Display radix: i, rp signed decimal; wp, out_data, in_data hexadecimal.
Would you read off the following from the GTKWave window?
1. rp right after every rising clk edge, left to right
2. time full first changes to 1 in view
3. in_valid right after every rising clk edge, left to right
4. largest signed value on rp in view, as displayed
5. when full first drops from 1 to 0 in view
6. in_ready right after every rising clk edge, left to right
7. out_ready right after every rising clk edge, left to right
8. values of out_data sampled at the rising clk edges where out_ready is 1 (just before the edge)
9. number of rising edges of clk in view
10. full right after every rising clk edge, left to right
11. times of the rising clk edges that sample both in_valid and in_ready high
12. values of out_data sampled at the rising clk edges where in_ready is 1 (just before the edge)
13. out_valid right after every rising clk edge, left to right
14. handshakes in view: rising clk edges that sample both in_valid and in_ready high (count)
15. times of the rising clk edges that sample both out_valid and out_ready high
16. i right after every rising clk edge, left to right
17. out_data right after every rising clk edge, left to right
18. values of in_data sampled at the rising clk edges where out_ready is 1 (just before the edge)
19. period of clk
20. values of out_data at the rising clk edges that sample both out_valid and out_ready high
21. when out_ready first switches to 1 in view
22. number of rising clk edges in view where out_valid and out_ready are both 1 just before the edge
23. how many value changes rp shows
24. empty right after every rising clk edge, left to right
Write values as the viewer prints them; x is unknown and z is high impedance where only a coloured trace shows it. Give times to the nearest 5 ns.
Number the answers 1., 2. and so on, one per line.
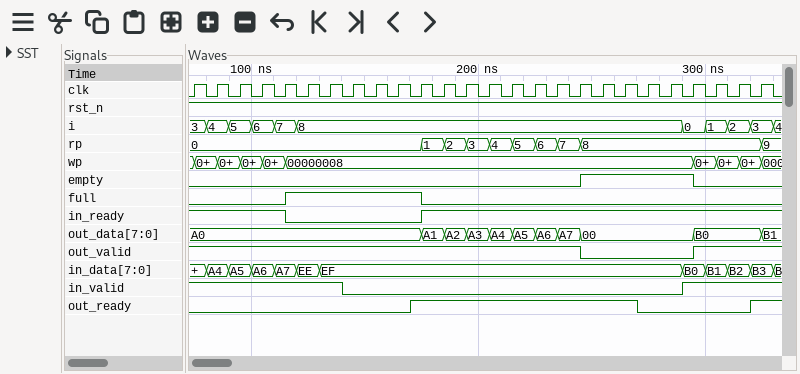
1. 0, 0, 0, 0, 0, 0, 0, 0, 0, 0, 1, 2, 3, 4, 5, 6, 7, 8, 8, 8, 8, 8, 8, 8, 8, 9
2. 115 ns
3. 1 1 1 1 1 1 1 0 0 0 0 0 0 0 0 0 0 0 0 0 0 0 1 1 1 1
4. 9
5. 175 ns
6. 1 1 1 1 0 0 0 0 0 0 1 1 1 1 1 1 1 1 1 1 1 1 1 1 1 1
7. 0 0 0 0 0 0 0 0 0 0 1 1 1 1 1 1 1 1 1 1 0 0 0 0 0 1
8. A0, A1, A2, A3, A4, A5, A6, A7, 00, 00, B0
9. 26
10. 0 0 0 0 1 1 1 1 1 1 0 0 0 0 0 0 0 0 0 0 0 0 0 0 0 0
11. 75 ns, 85 ns, 95 ns, 105 ns, 115 ns, 295 ns, 305 ns, 315 ns, 325 ns
12. A0, A0, A0, A0, A0, A1, A2, A3, A4, A5, A6, A7, 00, 00, 00, 00, 00, B0, B0, B0
13. 1 1 1 1 1 1 1 1 1 1 1 1 1 1 1 1 1 0 0 0 0 0 1 1 1 1
14. 9
15. 175 ns, 185 ns, 195 ns, 205 ns, 215 ns, 225 ns, 235 ns, 245 ns, 325 ns
16. 3, 4, 5, 6, 7, 8, 8, 8, 8, 8, 8, 8, 8, 8, 8, 8, 8, 8, 8, 8, 8, 8, 0, 1, 2, 3
17. A0, A0, A0, A0, A0, A0, A0, A0, A0, A0, A1, A2, A3, A4, A5, A6, A7, 00, 00, 00, 00, 00, B0, B0, B0, B1
18. EF, EF, EF, EF, EF, EF, EF, EF, EF, EF, B3
19. 10 ns
20. A0, A1, A2, A3, A4, A5, A6, A7, B0
21. 170 ns
22. 9
23. 9
24. 0 0 0 0 0 0 0 0 0 0 0 0 0 0 0 0 0 1 1 1 1 1 0 0 0 0
